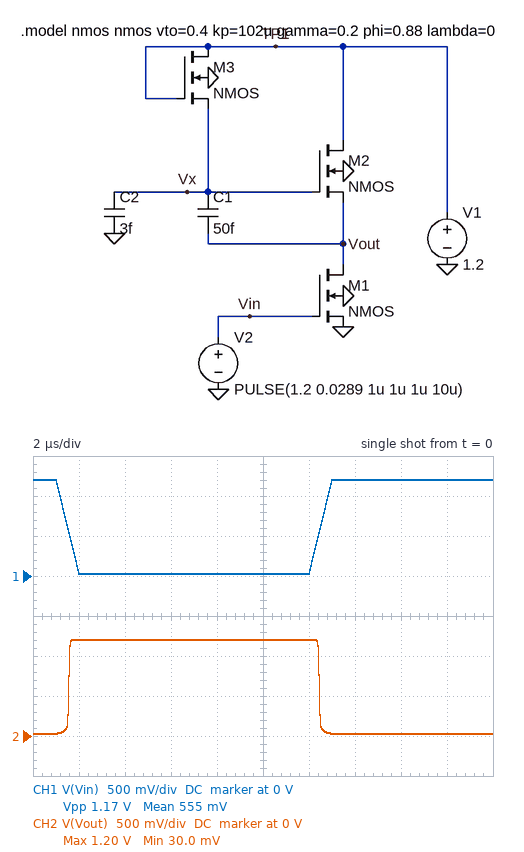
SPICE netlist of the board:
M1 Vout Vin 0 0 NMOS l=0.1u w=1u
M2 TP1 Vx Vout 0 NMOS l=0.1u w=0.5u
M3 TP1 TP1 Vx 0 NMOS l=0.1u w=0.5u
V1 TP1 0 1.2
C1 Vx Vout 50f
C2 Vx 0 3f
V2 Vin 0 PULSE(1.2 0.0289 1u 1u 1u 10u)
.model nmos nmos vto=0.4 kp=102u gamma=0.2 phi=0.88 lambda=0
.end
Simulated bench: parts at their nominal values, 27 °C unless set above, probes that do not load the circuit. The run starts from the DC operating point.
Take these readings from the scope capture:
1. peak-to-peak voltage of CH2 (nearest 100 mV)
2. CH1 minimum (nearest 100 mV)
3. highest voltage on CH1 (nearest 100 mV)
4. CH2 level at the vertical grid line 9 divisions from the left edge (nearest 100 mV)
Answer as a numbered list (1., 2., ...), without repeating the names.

1. 1.2 V
2. 0 V
3. 1.2 V
4. 0 V
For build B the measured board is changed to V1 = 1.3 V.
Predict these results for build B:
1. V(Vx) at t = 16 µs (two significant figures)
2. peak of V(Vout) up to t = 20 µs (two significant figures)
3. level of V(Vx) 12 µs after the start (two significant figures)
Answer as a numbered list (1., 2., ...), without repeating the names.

1. 830 mV
2. 1.3 V
3. 2.0 V
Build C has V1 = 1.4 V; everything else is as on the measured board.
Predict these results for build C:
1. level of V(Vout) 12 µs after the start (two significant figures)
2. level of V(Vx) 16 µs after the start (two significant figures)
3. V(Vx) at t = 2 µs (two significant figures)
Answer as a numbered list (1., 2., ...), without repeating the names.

1. 1.4 V
2. 920 mV
3. 2.2 V
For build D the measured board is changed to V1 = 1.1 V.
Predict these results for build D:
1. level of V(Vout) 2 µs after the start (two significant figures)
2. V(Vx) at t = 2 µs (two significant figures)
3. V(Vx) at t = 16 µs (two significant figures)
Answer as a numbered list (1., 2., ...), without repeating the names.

1. 1.1 V
2. 1.7 V
3. 640 mV
